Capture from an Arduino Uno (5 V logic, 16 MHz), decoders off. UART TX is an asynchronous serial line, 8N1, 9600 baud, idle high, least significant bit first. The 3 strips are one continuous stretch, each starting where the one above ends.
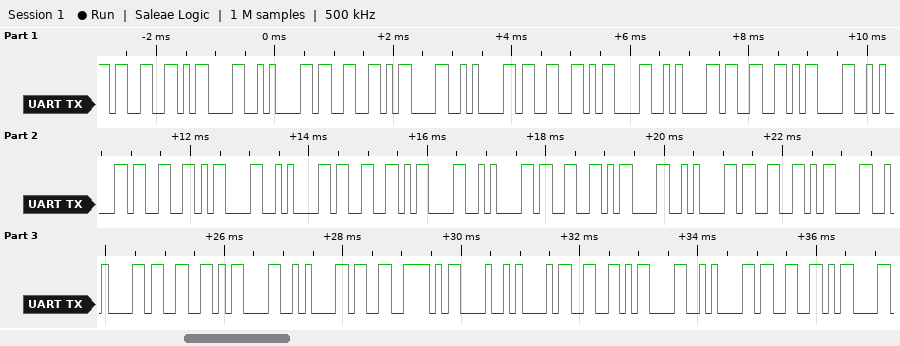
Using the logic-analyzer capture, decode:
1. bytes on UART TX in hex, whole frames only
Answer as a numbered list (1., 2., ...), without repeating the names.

1. 0x33 0x0D 0x0A 0x33 0x0D 0x0A 0x33 0x0D 0x0A 0x33 0x0D 0x0A 0x33 0x0D 0x0A 0x33 0x0D 0x0A 0x33 0x0D 0x0A 0x33 0x0D 0x0A 0x33 0x0D 0x0A 0x33 0x0D 0x0A 0x33 0x0D 0x0A 0x33 0x0D
